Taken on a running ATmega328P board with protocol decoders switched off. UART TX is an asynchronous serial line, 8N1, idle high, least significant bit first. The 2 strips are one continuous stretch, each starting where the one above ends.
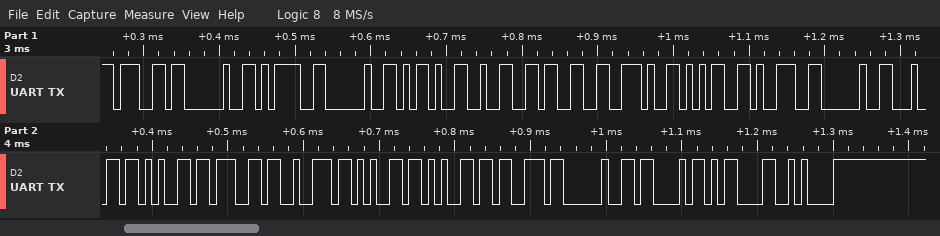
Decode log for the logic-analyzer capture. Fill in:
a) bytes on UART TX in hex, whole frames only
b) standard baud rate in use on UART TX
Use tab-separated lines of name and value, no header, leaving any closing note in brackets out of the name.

bytes on UART TX in hex, whole frames only	0x67 0x20 0x3D 0x20 0x2D 0x32 0x33 0x2E 0x35 0x39 0x20 0x64 0x65 0x67 0x72 0x65 0x65 0x73 0x20 0x43 0x0D 0x0A
standard baud rate in use on UART TX	115200 baud
